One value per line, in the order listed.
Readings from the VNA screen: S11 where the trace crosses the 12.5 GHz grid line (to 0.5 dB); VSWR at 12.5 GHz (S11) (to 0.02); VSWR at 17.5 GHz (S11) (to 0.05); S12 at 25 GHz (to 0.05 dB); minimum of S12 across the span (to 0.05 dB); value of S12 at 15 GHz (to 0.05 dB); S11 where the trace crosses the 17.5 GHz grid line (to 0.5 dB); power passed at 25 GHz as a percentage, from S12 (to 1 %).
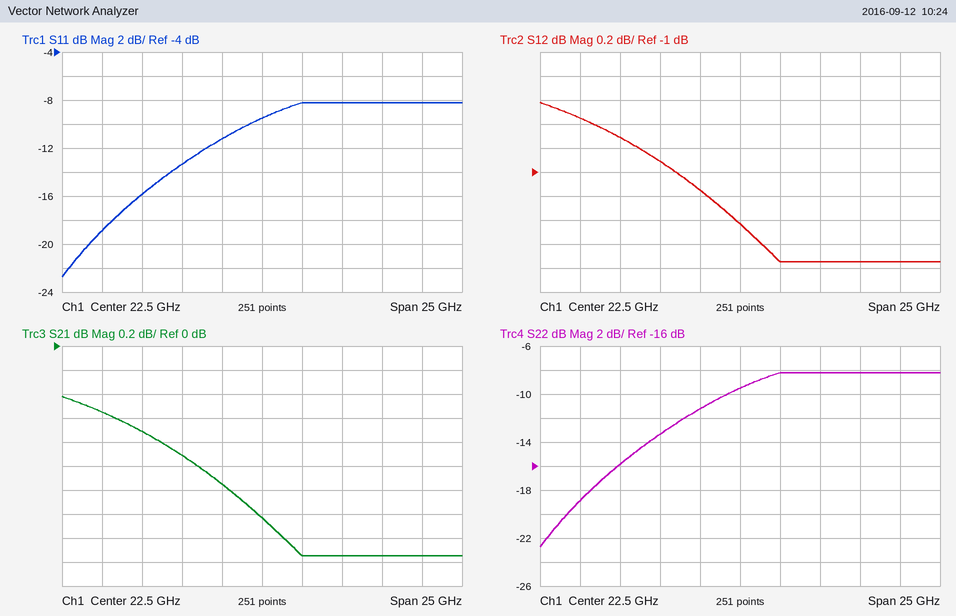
-19.0 dB
1.26
1.55
-1.75 dB
-1.75 dB
-0.70 dB
-13.5 dB
67 %
